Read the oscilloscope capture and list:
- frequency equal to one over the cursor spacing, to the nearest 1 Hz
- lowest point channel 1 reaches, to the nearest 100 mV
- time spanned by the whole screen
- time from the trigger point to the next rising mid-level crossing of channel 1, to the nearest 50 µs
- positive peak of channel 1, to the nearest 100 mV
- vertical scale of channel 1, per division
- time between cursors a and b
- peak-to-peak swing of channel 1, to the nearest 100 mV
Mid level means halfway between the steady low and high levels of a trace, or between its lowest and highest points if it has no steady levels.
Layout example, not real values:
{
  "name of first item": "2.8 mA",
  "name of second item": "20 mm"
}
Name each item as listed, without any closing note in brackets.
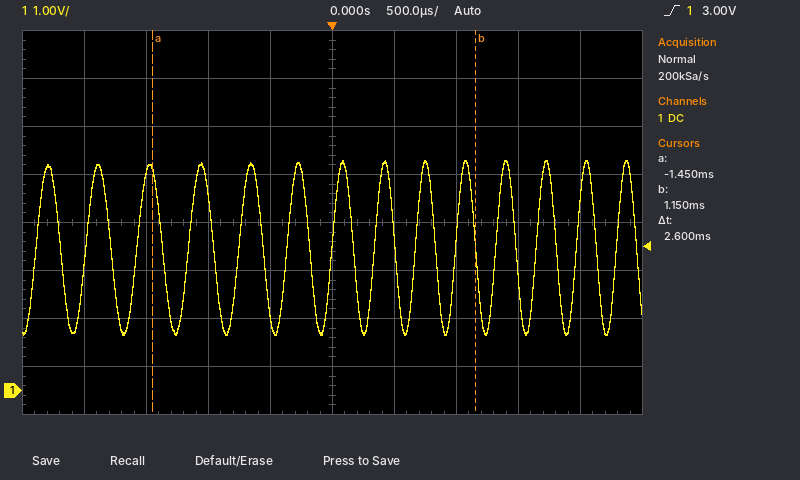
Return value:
{
  "frequency equal to one over the cursor spacing, to the nearest 1 Hz": "385 Hz",
  "lowest point channel 1 reaches, to the nearest 100 mV": "1.2 V",
  "time spanned by the whole screen": "5 ms",
  "time from the trigger point to the next rising mid-level crossing of channel 1, to the nearest 50 µs": "350 µs",
  "positive peak of channel 1, to the nearest 100 mV": "4.8 V",
  "vertical scale of channel 1, per division": "1 V",
  "time between cursors a and b": "2.6 ms",
  "peak-to-peak swing of channel 1, to the nearest 100 mV": "3.6 V"
}
